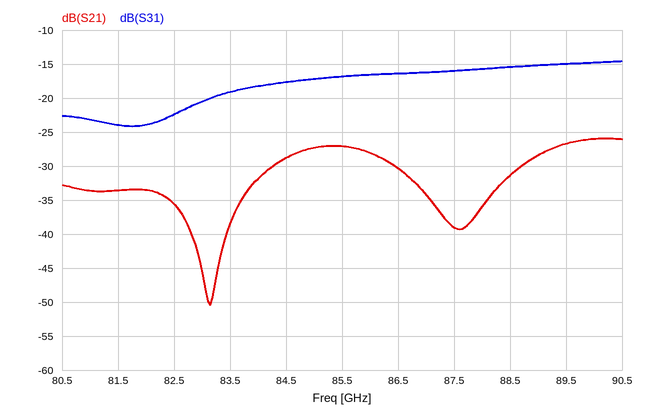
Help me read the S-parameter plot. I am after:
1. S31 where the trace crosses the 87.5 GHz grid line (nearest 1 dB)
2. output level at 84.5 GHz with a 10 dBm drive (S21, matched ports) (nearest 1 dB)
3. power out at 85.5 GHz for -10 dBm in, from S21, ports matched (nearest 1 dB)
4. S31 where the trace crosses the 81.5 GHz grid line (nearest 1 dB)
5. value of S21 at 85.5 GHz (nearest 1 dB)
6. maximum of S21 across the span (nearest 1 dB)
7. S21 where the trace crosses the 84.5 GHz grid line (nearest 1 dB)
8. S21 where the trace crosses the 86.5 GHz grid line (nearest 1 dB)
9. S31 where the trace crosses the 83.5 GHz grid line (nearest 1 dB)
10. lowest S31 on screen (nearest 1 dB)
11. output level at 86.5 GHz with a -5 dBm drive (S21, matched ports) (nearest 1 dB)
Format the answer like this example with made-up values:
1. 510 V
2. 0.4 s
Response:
1. -16 dB
2. -19 dBm
3. -37 dBm
4. -24 dB
5. -27 dB
6. -26 dB
7. -29 dB
8. -30 dB
9. -19 dB
10. -24 dB
11. -35 dBm
